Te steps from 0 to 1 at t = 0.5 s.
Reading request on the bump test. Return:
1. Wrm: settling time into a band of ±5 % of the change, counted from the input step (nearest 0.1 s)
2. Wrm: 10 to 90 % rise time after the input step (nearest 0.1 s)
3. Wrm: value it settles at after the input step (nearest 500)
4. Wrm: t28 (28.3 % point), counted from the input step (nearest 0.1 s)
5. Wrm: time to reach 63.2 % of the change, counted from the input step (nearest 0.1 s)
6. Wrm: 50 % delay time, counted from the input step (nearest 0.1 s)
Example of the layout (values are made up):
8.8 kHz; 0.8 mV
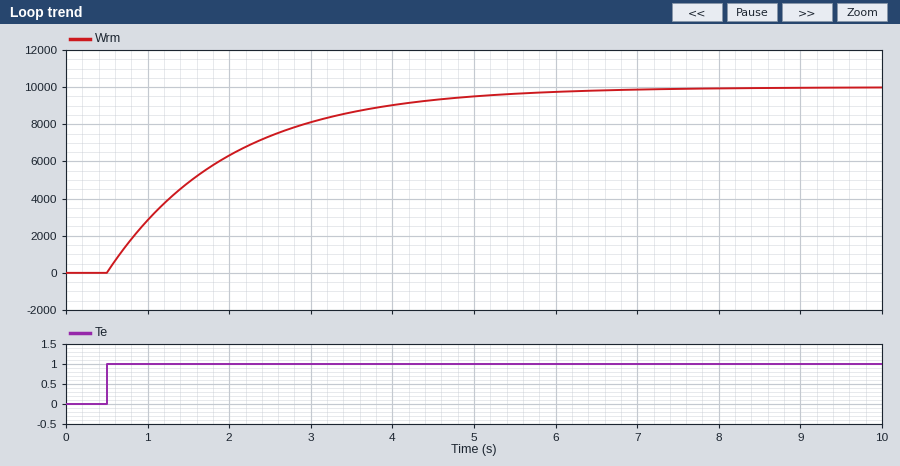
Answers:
4.5 s; 3.3 s; 10000; 0.5 s; 1.5 s; 1.0 s
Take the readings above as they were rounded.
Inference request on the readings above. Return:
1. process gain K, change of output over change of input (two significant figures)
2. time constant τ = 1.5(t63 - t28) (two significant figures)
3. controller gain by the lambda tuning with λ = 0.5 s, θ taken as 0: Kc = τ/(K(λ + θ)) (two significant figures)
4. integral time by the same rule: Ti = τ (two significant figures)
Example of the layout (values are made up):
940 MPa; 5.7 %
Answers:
10000; 1.5 s; 0.00030; 1.5 s
